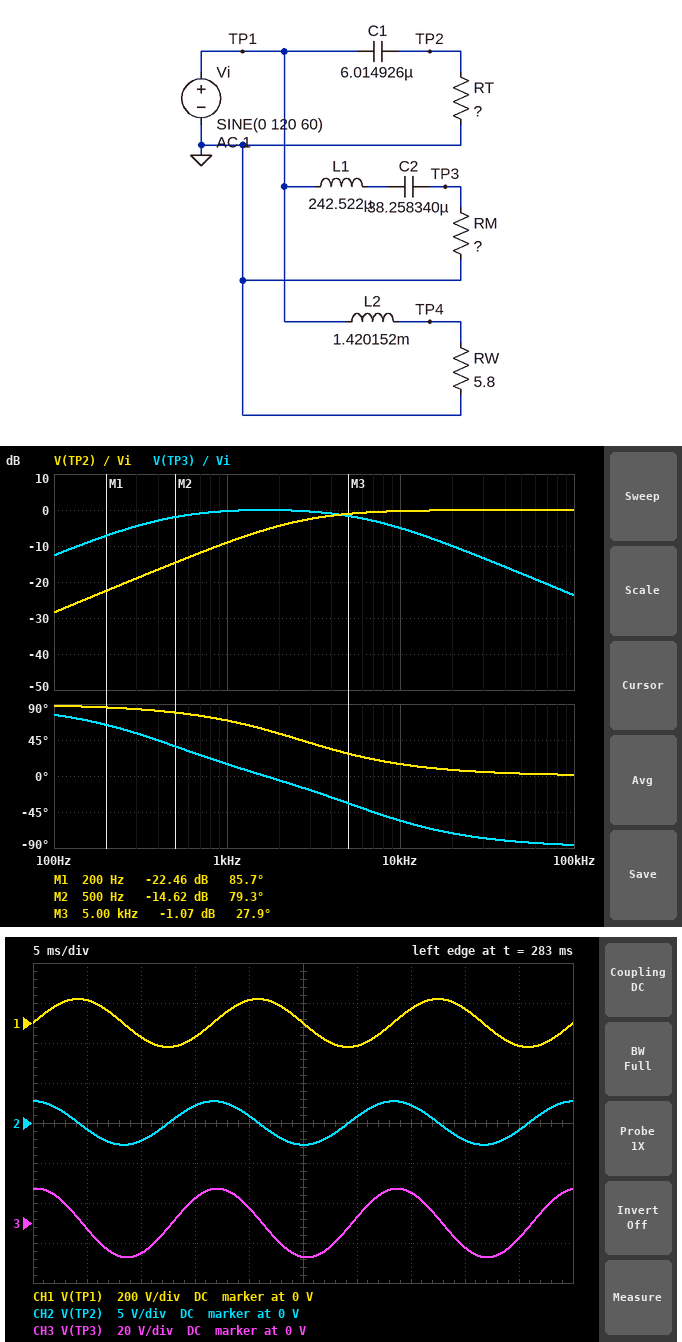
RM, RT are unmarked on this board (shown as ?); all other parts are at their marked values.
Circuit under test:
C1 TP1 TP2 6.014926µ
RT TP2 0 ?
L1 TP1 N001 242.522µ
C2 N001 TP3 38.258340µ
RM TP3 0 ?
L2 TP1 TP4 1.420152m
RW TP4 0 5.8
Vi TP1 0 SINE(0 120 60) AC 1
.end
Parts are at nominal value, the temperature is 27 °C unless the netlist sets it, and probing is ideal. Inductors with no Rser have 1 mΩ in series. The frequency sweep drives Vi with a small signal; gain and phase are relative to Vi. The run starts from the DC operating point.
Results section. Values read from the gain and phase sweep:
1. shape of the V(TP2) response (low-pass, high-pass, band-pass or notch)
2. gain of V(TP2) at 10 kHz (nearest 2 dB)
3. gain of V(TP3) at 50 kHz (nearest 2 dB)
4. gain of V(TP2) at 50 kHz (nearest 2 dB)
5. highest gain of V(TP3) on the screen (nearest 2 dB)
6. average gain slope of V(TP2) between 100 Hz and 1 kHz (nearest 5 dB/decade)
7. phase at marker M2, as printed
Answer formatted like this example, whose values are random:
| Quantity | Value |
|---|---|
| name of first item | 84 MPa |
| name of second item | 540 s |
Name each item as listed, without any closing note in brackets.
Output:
| Quantity | Value |
|---|---|
| shape of the V(TP2) response | high-pass |
| gain of V(TP2) at 10 kHz | 0 dB |
| gain of V(TP3) at 50 kHz | -18 dB |
| gain of V(TP2) at 50 kHz | 0 dB |
| highest gain of V(TP3) on the screen | 0 dB |
| average gain slope of V(TP2) between 100 Hz and 1 kHz | 20 dB/decade |
| phase at marker M2, as printed | 79.3 deg |
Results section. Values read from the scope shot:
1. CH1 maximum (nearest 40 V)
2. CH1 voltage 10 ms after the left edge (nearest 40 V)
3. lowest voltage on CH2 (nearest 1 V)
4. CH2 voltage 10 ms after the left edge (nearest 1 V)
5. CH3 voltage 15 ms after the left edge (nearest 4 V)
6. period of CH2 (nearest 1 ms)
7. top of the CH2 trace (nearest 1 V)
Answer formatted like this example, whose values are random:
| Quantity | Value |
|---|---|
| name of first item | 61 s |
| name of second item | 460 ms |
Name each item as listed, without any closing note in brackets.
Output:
| Quantity | Value |
|---|---|
| CH1 maximum | 120 V |
| CH1 voltage 10 ms after the left edge | -80 V |
| lowest voltage on CH2 | -3 V |
| CH2 voltage 10 ms after the left edge | -2 V |
| CH3 voltage 15 ms after the left edge | 12 V |
| period of CH2 | 17 ms |
| top of the CH2 trace | 3 V |
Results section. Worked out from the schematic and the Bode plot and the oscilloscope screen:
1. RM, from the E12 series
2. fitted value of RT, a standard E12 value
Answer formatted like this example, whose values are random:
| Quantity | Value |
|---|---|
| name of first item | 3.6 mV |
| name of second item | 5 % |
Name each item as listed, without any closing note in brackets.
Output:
| Quantity | Value |
|---|---|
| RM, from the E12 series | 10 Ω |
| fitted value of RT, a standard E12 value | 10 Ω |
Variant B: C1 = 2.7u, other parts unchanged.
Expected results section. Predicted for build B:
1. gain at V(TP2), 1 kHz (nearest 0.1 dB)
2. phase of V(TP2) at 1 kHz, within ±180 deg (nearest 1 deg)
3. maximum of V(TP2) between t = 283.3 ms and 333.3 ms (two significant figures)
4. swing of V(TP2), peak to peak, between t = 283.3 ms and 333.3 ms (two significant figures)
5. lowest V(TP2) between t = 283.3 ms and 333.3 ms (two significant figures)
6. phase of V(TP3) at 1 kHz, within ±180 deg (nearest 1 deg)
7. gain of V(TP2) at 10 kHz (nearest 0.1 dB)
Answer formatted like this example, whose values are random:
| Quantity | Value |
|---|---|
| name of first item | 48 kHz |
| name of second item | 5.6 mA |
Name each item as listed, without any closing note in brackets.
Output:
| Quantity | Value |
|---|---|
| gain at V(TP2), 1 kHz | -15.5 dB |
| phase of V(TP2) at 1 kHz, within ±180 deg | 80 deg |
| maximum of V(TP2) between t = 283.3 ms and 333.3 ms | 1.2 V |
| swing of V(TP2), peak to peak, between t = 283.3 ms and 333.3 ms | 2.4 V |
| lowest V(TP2) between t = 283.3 ms and 333.3 ms | -1.2 V |
| phase of V(TP3) at 1 kHz, within ±180 deg | 15 deg |
| gain of V(TP2) at 10 kHz | -1.3 dB |
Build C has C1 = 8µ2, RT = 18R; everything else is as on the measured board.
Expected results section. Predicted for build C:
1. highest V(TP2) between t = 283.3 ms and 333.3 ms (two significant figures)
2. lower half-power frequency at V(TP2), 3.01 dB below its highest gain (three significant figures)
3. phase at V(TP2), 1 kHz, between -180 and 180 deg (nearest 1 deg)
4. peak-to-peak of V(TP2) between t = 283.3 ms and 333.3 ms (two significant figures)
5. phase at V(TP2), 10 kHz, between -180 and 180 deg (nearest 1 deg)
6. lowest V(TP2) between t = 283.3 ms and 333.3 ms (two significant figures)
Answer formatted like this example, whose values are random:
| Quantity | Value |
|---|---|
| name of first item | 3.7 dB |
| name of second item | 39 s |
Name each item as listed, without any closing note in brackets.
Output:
| Quantity | Value |
|---|---|
| highest V(TP2) between t = 283.3 ms and 333.3 ms | 6.7 V |
| lower half-power frequency at V(TP2), 3.01 dB below its highest gain | 1.08 kHz |
| phase at V(TP2), 1 kHz, between -180 and 180 deg | 47 deg |
| peak-to-peak of V(TP2) between t = 283.3 ms and 333.3 ms | 13 V |
| phase at V(TP2), 10 kHz, between -180 and 180 deg | 6 deg |
| lowest V(TP2) between t = 283.3 ms and 333.3 ms | -6.7 V |
